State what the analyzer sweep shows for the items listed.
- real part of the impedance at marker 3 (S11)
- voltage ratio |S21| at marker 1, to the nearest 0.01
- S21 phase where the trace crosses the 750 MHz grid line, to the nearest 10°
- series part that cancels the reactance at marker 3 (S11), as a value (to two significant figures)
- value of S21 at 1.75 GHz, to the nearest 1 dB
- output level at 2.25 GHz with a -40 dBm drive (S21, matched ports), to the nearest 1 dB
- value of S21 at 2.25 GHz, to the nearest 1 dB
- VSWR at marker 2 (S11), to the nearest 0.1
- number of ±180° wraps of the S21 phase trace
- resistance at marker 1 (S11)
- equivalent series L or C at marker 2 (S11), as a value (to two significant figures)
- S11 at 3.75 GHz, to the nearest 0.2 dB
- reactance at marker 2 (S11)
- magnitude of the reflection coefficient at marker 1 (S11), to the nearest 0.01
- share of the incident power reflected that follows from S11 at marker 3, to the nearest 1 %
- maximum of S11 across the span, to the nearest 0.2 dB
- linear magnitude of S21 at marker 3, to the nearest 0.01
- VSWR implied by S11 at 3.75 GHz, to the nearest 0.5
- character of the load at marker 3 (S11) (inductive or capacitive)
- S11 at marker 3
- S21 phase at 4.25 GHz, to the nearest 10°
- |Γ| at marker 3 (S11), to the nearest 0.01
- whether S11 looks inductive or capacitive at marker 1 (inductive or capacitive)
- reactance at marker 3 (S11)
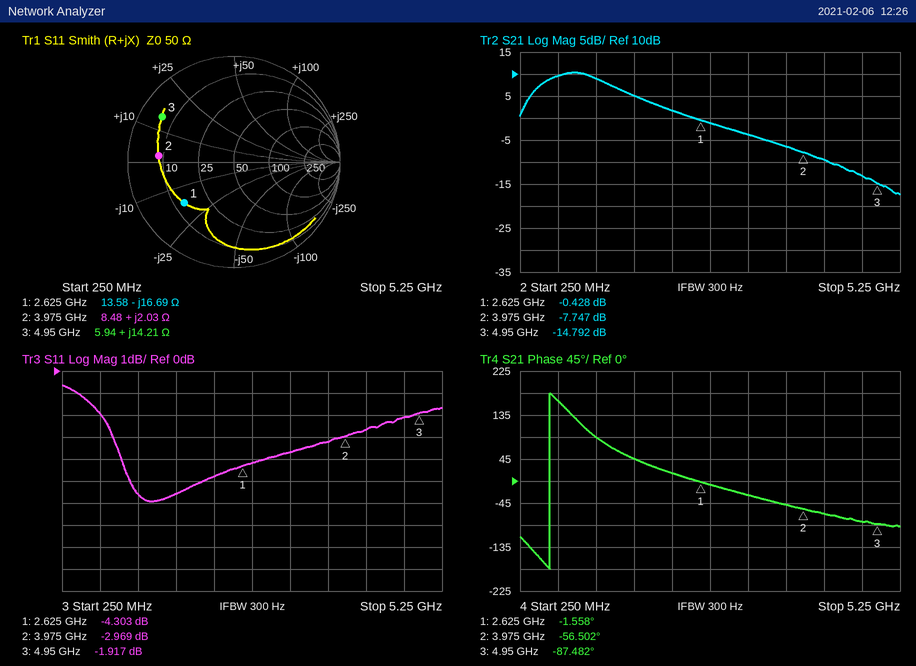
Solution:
5.94 Ω
0.95
160°
2.3 pF
5 dB
-38 dBm
2 dB
5.9
1
13.58 Ω
81 pH
-3.2 dB
+2.03 Ω
0.61
64 %
-0.6 dB
0.18
5.5
inductive
-1.917 dB
-70°
0.80
capacitive
+14.21 Ω
